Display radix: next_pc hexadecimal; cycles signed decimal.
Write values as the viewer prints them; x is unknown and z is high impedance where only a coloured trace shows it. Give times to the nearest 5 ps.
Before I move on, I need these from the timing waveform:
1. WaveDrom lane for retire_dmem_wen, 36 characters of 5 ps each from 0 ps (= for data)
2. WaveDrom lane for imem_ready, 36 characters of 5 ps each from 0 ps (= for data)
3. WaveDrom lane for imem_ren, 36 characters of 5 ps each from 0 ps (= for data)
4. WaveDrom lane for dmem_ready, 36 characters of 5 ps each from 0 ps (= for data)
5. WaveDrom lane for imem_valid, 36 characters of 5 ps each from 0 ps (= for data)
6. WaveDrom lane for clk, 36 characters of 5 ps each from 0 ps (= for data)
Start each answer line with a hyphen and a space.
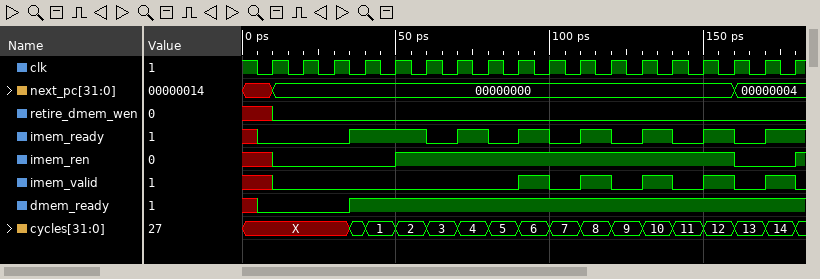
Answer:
- {name: 'retire_dmem_wen', wave: 'x.0.................................'}
- {name: 'imem_ready', wave: 'x0.....1....0.1.0.1.0.1.0.1.0.1.0.1.'}
- {name: 'imem_ren', wave: 'x.0.......1.....................0...'}
- {name: 'dmem_ready', wave: 'x0.....1............................'}
- {name: 'imem_valid', wave: 'x.0...............1.0.1.0.1.0.1.0.1.'}
- {name: 'clk', wave: '101010101010101010101010101010101010'}
